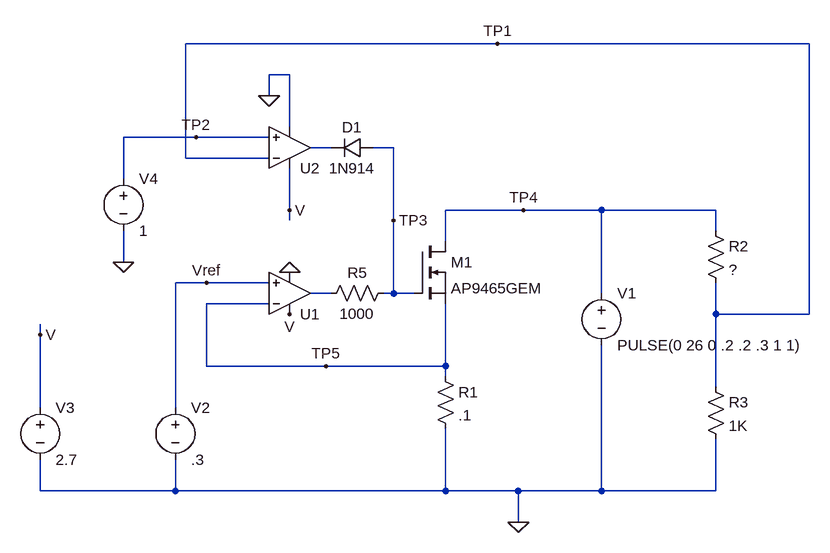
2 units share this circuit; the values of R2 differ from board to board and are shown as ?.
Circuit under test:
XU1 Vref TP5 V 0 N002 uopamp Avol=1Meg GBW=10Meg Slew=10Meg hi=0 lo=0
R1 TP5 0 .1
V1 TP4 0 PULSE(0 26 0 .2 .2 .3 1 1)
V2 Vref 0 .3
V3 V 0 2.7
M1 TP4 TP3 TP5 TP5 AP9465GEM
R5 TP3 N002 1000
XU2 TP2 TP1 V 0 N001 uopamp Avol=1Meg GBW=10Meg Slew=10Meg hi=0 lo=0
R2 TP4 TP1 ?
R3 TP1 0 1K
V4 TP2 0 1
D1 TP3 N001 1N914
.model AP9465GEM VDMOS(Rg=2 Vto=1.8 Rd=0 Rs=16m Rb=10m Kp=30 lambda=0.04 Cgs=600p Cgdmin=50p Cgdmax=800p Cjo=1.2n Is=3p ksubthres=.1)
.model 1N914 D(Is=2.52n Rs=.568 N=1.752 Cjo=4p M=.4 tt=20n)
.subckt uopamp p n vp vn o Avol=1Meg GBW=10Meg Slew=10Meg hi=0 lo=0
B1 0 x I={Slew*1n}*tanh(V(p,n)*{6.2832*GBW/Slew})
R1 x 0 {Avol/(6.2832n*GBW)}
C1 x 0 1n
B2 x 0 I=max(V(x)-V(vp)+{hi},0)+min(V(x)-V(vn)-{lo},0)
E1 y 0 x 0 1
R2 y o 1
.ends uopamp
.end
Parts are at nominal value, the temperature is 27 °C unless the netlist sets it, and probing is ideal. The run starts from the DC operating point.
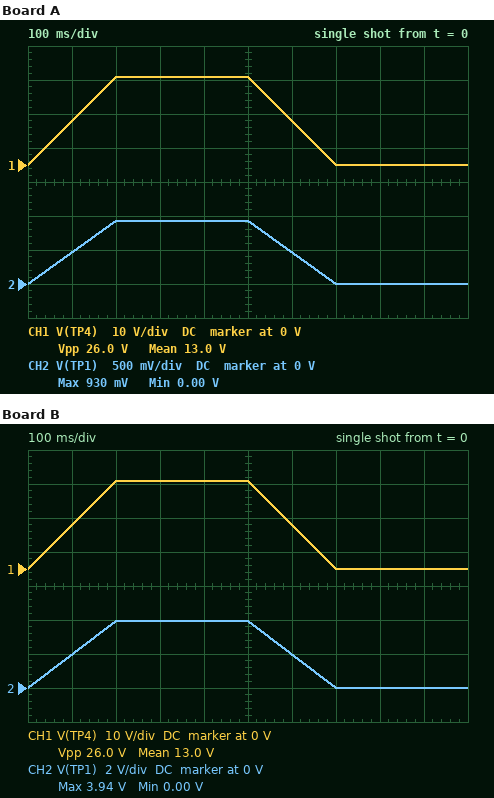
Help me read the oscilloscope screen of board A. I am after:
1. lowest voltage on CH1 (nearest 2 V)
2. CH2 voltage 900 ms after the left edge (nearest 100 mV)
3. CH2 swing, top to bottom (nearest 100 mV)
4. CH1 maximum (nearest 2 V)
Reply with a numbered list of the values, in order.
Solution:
1. 0 V
2. 0 V
3. 900 mV
4. 26 V
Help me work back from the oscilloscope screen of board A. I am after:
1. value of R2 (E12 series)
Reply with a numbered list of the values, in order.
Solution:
1. 27 kΩ
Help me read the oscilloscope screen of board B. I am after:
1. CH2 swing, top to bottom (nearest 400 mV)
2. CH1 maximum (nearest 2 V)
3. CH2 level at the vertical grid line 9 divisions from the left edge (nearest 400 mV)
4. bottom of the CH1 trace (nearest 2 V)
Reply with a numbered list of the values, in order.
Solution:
1. 4.0 V
2. 26 V
3. 0 V
4. 0 V
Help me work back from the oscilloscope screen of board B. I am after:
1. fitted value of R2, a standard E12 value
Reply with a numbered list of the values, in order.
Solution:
1. 5.6 kΩ
